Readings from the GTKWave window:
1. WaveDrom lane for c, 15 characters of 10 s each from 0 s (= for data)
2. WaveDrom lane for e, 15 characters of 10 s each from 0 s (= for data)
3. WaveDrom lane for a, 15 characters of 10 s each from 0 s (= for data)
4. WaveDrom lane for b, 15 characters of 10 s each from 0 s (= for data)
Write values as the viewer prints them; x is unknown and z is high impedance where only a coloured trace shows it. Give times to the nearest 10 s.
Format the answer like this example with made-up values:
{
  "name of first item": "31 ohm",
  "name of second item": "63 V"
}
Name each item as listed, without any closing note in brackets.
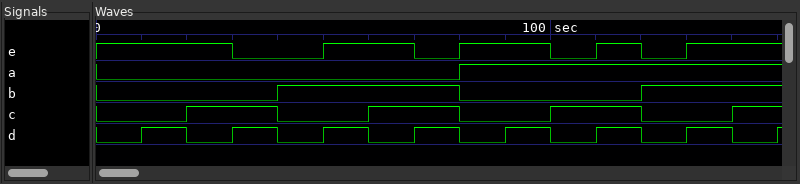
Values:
{
  "WaveDrom lane for c, 15 characters of 10 s each from 0 s": "{name: 'c', wave: '0.1.0.1.0.1.0.1'}",
  "WaveDrom lane for e, 15 characters of 10 s each from 0 s": "{name: 'e', wave: '1..0.1.01.0101.'}",
  "WaveDrom lane for a, 15 characters of 10 s each from 0 s": "{name: 'a', wave: '0.......1......'}",
  "WaveDrom lane for b, 15 characters of 10 s each from 0 s": "{name: 'b', wave: '0...1...0...1..'}"
}
